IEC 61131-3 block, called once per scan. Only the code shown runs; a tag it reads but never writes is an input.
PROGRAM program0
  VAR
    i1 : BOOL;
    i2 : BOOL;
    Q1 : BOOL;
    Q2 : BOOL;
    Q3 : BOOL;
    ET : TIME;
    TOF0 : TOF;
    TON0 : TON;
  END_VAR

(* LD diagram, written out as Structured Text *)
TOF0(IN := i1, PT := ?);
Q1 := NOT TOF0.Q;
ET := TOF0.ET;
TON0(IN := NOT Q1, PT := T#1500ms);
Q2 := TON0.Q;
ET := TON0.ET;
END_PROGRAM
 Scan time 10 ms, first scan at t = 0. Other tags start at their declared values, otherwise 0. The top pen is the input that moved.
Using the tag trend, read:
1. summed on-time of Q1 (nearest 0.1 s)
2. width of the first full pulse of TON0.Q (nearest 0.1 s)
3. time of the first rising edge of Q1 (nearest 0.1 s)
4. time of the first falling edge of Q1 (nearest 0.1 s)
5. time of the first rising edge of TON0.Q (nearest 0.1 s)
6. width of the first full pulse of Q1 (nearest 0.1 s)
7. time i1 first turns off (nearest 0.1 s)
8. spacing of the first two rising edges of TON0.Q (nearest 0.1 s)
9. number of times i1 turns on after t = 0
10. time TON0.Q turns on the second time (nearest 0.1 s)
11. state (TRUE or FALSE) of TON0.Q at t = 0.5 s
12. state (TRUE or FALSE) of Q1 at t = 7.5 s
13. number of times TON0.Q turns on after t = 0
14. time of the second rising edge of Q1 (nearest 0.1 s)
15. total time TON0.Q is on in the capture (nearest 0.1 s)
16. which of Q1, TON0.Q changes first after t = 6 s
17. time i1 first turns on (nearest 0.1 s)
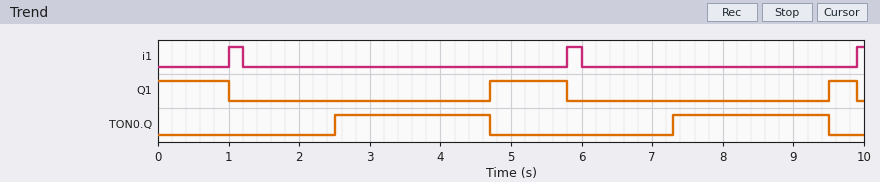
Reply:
2.5 s
2.2 s
4.7 s
1.0 s
2.5 s
1.1 s
1.2 s
4.8 s
3
7.3 s
FALSE
FALSE
2
9.5 s
4.4 s
TON0.Q
1.0 s
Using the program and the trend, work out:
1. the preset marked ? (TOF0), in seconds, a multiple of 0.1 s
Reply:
3.5 s
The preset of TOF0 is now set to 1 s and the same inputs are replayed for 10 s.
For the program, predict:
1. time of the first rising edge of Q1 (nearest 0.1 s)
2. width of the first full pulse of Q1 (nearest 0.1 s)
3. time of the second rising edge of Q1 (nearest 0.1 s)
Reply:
2.2 s
3.6 s
7.0 s
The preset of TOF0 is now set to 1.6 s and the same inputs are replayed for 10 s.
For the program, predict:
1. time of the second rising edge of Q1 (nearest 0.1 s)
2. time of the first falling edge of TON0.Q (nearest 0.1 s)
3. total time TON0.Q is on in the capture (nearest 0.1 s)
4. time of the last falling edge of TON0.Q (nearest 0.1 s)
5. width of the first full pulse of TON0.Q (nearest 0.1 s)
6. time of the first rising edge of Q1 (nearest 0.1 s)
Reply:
7.6 s
2.8 s
0.6 s
7.6 s
0.3 s
2.8 s
